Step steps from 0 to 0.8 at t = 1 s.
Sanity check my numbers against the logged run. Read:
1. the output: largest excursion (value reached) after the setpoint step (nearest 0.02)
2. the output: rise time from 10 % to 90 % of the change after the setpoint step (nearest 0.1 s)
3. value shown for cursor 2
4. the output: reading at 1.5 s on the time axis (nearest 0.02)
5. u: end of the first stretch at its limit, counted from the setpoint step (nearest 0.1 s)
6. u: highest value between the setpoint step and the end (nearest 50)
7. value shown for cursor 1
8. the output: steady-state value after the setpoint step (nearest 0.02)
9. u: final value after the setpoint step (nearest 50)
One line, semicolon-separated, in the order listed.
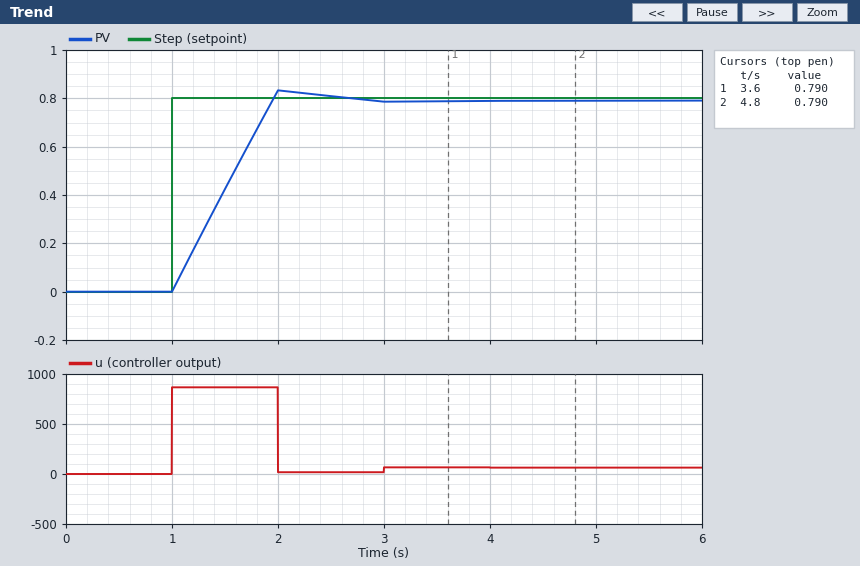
0.84; 0.8 s; 0.790; 0.42; 1.0 s; 850; 0.790; 0.80; 50
